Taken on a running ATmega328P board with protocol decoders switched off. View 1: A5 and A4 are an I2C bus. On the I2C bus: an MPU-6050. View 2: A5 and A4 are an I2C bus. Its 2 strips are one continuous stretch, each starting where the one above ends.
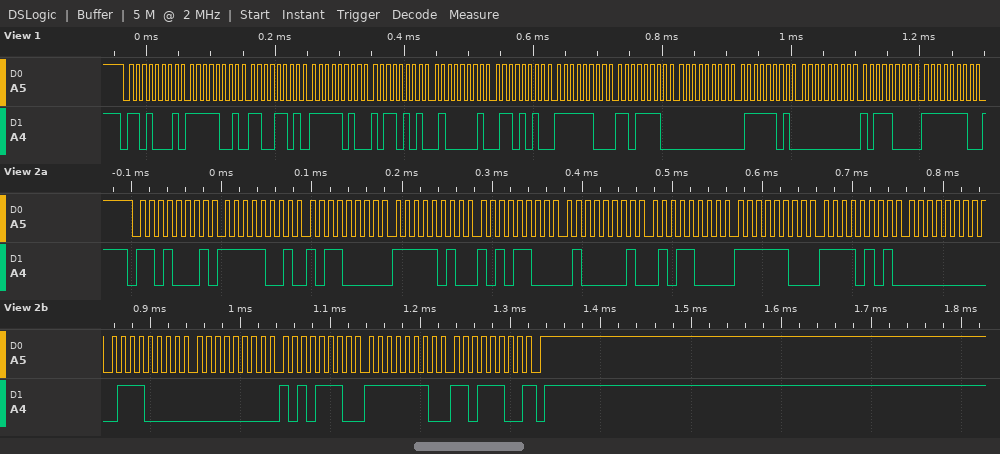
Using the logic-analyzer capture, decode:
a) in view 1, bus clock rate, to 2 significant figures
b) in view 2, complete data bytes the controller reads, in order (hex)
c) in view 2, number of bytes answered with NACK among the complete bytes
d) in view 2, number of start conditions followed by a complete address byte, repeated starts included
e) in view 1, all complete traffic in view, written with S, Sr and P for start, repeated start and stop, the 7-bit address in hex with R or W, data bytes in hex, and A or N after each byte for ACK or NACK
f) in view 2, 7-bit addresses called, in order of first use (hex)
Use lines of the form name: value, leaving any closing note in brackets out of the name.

in view 1, bus clock rate, to 2 significant figures: 100 kHz
in view 2, complete data bytes the controller reads, in order: F9 B0 FA AC 41 58 FC F5 00 70 00 AE FE DC
in view 2, number of bytes answered with NACK among the complete bytes: 1
in view 2, number of start conditions followed by a complete address byte, repeated starts included: 1
in view 1, all complete traffic in view, written with S, Sr and P for start, repeated start and stop, the 7-bit address in hex with R or W, data bytes in hex, and A or N after each byte for ACK or NACK: S 68R A F9 A CD A FA A B5 A 41 A 6A A FC A DE A 00 A 7D A 00 A B8 A FE A
in view 2, 7-bit addresses called, in order of first use: 0x68
